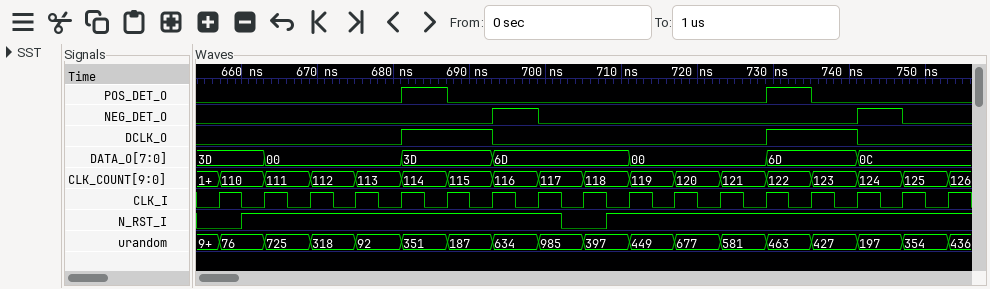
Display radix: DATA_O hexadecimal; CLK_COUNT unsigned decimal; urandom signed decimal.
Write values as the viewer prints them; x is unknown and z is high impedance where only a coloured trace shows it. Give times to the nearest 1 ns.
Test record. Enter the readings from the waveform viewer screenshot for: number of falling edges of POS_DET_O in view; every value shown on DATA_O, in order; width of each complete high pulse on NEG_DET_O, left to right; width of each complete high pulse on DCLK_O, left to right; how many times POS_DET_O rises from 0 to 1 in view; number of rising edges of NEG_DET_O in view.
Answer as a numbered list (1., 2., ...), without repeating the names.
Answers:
1. 2
2. 3D, 00, 3D, 6D, 00, 6D, 0C
3. 6 ns, 6 ns
4. 12 ns, 12 ns
5. 2
6. 2
